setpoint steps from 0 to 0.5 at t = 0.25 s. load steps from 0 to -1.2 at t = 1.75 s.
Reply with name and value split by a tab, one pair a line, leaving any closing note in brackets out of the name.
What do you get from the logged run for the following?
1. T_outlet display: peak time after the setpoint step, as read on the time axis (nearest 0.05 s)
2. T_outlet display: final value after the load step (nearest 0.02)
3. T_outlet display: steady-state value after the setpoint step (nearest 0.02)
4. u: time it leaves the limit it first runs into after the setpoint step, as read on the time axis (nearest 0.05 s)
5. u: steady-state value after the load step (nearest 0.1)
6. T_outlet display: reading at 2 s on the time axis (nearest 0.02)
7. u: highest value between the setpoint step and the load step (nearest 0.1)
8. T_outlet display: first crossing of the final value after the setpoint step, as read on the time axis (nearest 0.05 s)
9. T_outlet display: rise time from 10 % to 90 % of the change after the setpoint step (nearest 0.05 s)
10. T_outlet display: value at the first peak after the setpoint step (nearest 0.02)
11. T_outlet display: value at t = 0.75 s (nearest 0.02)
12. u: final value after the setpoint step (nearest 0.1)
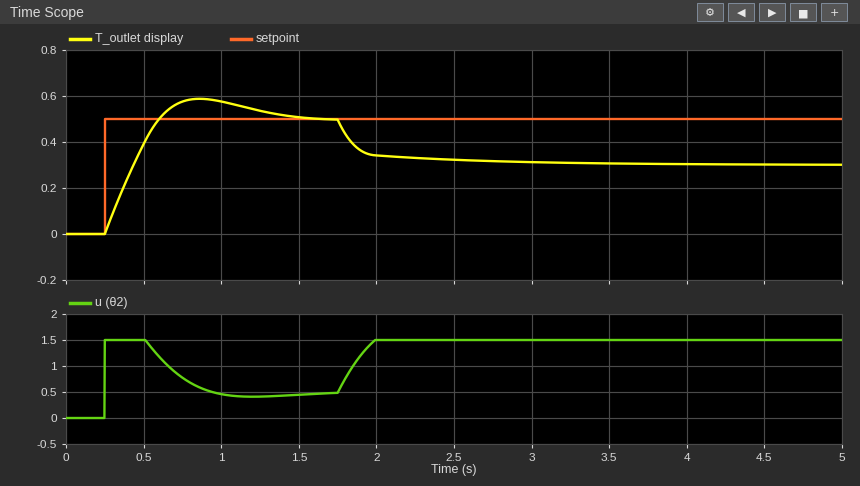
T_outlet display: peak time after the setpoint step, as read on the time axis	0.85 s
T_outlet display: final value after the load step	0.30
T_outlet display: steady-state value after the setpoint step	0.50
u: time it leaves the limit it first runs into after the setpoint step, as read on the time axis	0.50 s
u: steady-state value after the load step	1.5
T_outlet display: reading at 2 s on the time axis	0.34
u: highest value between the setpoint step and the load step	1.5
T_outlet display: first crossing of the final value after the setpoint step, as read on the time axis	0.60 s
T_outlet display: rise time from 10 % to 90 % of the change after the setpoint step	0.25 s
T_outlet display: value at the first peak after the setpoint step	0.58
T_outlet display: value at t = 0.75 s	0.58
u: final value after the setpoint step	0.5
